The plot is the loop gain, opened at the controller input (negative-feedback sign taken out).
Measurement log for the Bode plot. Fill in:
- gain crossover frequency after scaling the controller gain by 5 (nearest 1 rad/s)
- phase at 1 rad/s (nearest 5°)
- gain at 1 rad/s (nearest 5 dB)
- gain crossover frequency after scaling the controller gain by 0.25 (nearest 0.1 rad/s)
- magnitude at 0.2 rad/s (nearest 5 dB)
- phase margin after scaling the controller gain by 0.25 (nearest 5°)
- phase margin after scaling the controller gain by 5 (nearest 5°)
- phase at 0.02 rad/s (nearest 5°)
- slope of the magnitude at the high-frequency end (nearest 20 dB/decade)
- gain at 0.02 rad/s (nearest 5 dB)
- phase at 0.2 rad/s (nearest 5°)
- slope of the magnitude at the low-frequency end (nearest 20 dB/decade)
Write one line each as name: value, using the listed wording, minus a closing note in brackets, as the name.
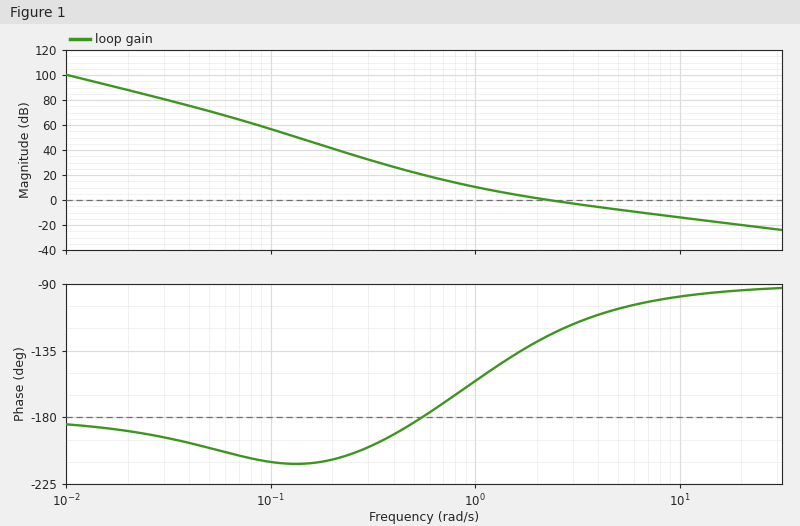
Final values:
gain crossover frequency after scaling the controller gain by 5: 10 rad/s
phase at 1 rad/s: -155°
gain at 1 rad/s: 10 dB
gain crossover frequency after scaling the controller gain by 0.25: 0.9 rad/s
magnitude at 0.2 rad/s: 40 dB
phase margin after scaling the controller gain by 0.25: 20°
phase margin after scaling the controller gain by 5: 80°
phase at 0.02 rad/s: -190°
slope of the magnitude at the high-frequency end: -20 dB/decade
gain at 0.02 rad/s: 90 dB
phase at 0.2 rad/s: -210°
slope of the magnitude at the low-frequency end: -40 dB/decade
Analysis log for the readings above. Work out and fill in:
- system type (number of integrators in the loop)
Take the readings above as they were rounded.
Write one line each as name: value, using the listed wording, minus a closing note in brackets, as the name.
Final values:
system type: 2
